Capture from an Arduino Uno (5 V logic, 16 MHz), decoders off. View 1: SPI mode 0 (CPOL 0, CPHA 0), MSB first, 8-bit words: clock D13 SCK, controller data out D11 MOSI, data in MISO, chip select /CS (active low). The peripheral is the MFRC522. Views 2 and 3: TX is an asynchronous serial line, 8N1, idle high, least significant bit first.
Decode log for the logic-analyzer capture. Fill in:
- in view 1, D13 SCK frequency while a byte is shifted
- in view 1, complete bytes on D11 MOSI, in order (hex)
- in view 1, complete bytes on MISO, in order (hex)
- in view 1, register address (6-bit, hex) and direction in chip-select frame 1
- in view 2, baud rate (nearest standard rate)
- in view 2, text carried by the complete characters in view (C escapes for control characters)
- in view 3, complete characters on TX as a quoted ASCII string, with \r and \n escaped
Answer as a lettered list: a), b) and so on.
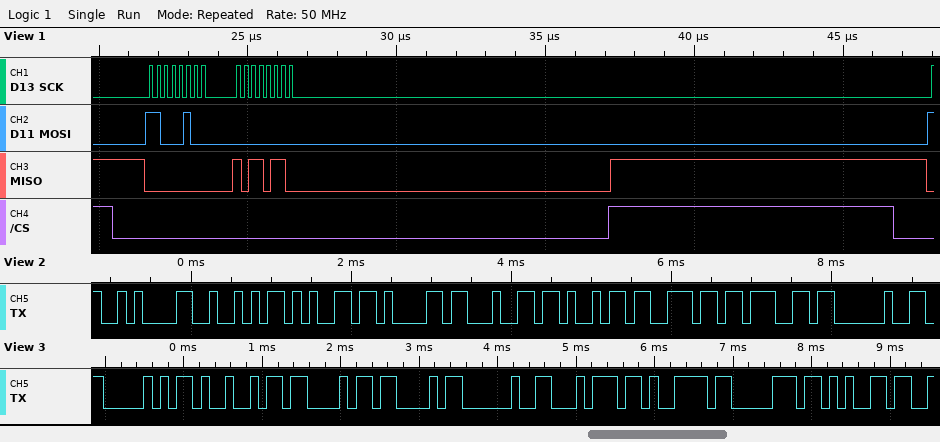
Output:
a) 4 MHz
b) 0xC4 0x00
c) 0x00 0xB6
d) 0x22 read
e) 9600 baud
f) "\nReading "
g) "PICC type"
